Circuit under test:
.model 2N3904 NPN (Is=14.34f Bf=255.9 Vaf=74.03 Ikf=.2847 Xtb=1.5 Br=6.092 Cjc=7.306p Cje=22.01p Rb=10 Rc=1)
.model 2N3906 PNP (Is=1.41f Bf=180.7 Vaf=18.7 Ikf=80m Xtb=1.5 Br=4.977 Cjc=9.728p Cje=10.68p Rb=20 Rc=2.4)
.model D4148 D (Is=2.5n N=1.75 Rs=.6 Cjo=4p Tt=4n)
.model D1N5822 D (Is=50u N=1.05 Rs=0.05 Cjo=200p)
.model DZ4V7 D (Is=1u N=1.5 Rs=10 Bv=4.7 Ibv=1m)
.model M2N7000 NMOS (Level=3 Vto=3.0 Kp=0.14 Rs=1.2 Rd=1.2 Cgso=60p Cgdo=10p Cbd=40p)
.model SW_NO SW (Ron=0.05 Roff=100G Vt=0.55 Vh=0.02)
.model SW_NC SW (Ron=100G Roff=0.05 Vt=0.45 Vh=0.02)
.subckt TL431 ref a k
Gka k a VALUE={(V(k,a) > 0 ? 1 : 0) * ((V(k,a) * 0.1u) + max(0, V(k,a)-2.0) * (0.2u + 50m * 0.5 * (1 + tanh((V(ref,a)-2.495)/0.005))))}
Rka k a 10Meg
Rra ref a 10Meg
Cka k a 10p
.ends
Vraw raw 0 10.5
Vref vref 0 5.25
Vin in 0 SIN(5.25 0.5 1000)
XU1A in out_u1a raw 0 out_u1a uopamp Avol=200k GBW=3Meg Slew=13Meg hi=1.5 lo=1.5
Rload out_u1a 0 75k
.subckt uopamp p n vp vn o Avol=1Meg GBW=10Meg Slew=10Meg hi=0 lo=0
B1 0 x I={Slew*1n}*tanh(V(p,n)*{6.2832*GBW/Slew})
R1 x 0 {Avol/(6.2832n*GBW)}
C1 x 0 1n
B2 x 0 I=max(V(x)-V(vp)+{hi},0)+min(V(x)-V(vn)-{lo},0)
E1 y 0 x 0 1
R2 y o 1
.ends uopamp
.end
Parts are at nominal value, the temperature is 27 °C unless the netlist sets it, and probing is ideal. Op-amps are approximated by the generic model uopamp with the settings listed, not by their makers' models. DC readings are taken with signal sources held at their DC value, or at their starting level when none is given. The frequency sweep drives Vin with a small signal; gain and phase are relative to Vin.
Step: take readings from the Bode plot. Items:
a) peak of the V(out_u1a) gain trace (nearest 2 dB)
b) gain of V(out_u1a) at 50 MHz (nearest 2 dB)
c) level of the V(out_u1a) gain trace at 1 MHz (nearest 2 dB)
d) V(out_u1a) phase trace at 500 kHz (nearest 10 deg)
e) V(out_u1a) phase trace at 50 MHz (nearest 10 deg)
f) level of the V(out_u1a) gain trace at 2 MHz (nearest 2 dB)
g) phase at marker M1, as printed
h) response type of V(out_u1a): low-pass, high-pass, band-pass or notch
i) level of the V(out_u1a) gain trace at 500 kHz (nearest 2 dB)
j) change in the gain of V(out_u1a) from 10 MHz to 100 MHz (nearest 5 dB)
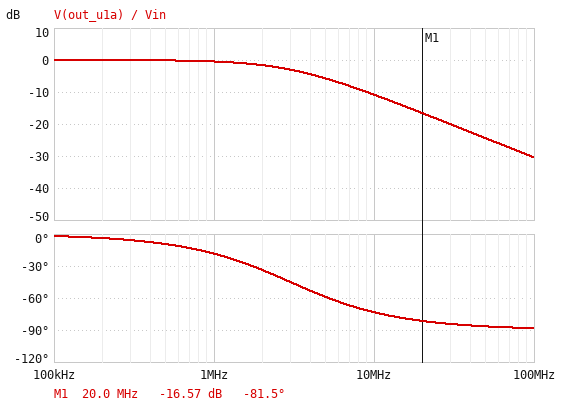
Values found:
0 dB
-24 dB
0 dB
-10 deg
-90 deg
-2 dB
-81.5 deg
low-pass
0 dB
-20 dB
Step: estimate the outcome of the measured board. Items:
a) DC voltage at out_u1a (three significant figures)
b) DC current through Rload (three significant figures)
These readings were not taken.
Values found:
5.25 V
70.0 µA
